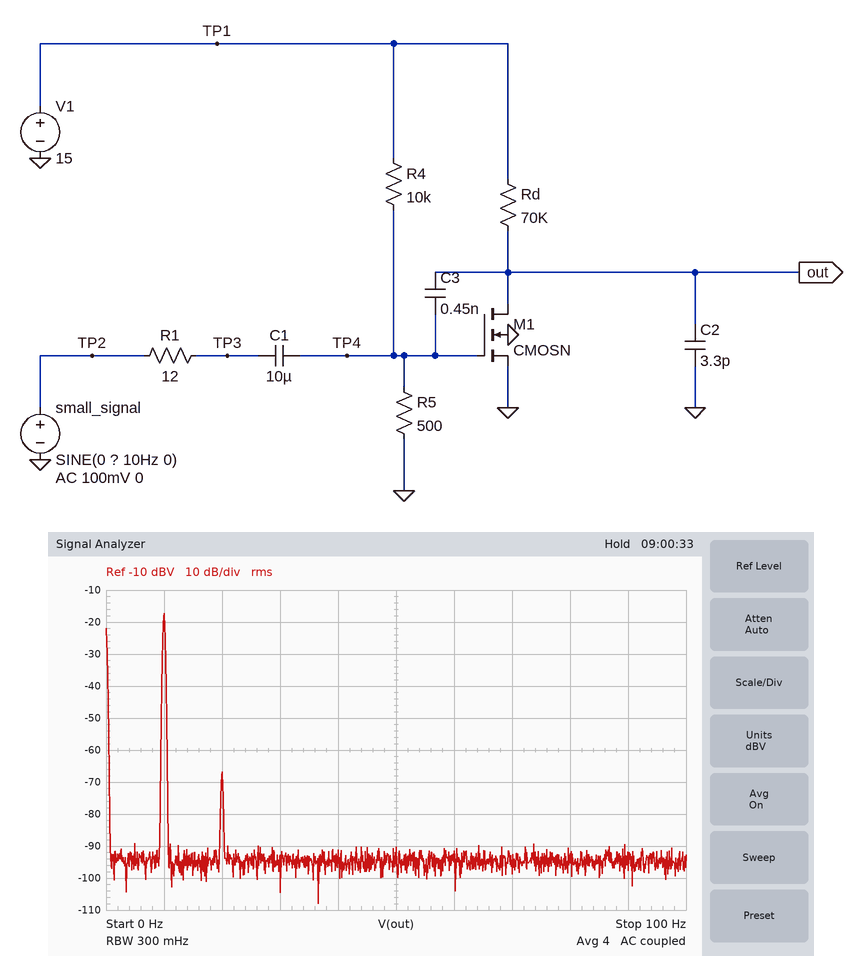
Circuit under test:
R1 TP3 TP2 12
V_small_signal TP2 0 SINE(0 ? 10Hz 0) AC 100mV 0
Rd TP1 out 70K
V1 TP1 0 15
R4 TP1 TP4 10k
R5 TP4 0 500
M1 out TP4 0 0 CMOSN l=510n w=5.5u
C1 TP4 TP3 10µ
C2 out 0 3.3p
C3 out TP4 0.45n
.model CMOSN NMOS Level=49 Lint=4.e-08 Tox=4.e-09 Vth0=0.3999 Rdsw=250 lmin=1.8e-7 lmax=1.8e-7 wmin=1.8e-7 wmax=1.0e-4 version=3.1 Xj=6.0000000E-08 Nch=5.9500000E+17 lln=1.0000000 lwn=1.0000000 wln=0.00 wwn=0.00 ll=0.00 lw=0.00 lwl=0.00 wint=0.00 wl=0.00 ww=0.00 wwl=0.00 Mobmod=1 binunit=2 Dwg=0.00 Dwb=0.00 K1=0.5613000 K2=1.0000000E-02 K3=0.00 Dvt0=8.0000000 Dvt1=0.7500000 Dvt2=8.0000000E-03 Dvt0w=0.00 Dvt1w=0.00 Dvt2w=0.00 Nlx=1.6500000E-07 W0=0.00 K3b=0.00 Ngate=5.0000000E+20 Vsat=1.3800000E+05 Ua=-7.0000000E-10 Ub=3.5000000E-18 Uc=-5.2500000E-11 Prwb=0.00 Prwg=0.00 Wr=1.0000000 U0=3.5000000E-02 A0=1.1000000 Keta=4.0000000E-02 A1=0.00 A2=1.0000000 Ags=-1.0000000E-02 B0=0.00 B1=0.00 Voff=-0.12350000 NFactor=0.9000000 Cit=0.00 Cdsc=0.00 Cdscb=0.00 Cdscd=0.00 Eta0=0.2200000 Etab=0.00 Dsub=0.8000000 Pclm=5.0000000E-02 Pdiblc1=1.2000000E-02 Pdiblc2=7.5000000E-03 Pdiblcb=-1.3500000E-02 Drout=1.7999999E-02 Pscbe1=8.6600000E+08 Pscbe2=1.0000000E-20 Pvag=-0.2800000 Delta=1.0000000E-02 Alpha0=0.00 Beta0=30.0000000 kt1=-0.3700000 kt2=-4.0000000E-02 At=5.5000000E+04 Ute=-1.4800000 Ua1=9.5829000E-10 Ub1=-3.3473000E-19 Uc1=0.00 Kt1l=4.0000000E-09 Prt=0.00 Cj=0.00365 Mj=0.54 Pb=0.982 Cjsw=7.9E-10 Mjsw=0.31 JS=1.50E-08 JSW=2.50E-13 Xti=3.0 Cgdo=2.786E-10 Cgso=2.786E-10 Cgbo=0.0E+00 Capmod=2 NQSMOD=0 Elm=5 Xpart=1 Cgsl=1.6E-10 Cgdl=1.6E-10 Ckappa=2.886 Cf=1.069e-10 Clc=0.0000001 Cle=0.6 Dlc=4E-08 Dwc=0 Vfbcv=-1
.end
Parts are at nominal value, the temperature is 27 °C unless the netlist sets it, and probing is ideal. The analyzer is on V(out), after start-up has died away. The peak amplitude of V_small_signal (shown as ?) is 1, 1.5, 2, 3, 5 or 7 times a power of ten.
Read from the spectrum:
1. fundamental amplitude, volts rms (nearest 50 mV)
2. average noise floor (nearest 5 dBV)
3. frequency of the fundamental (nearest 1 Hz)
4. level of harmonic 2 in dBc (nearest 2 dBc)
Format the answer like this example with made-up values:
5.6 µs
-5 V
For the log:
150 mV
-95 dBV
10 Hz
-50 dBc
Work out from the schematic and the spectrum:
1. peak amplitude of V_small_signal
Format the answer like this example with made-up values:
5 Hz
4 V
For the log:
20 mV
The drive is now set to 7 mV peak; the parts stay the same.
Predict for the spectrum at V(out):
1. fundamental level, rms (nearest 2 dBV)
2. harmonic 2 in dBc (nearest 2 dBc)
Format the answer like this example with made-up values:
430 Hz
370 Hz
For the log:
-26 dBV
-58 dBc
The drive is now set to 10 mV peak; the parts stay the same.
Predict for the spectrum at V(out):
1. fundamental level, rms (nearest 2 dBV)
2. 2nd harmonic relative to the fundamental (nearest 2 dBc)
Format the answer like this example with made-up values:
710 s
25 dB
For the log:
-24 dBV
-56 dBc
